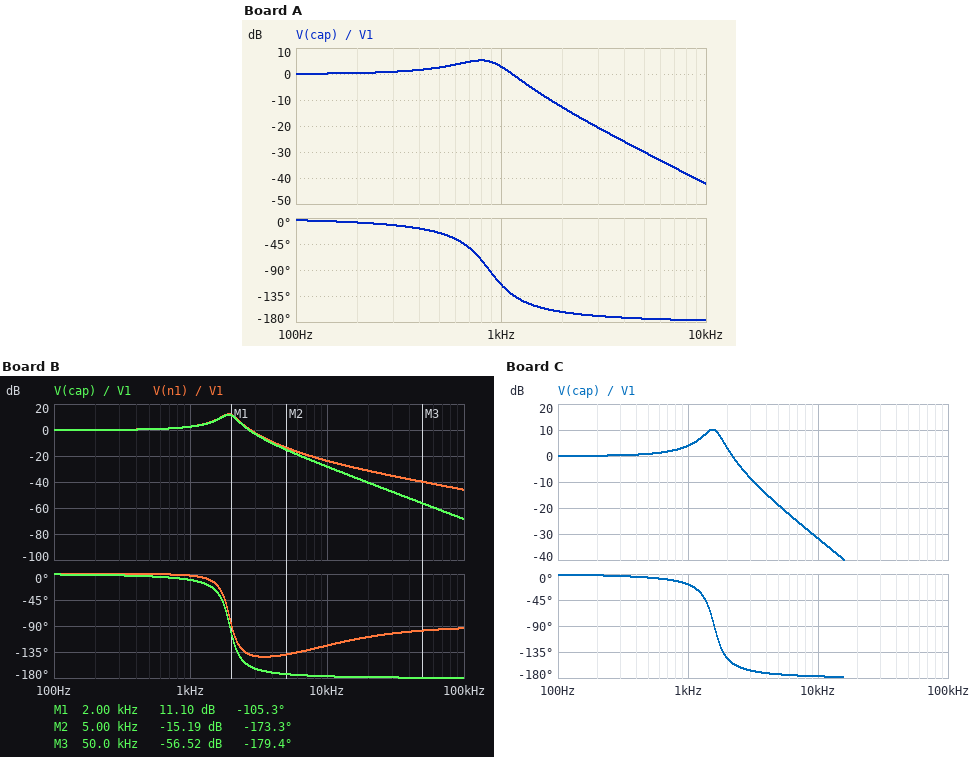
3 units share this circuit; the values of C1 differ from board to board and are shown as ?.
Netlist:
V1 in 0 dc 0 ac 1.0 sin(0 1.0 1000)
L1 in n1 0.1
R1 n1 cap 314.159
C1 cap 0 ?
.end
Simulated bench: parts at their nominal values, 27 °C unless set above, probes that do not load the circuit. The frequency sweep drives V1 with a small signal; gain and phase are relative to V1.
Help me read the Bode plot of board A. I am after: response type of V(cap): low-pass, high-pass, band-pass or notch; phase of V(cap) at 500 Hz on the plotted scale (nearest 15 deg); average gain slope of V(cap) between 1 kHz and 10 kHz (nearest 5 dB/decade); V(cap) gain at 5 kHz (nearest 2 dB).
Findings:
low-pass
-30 deg
-45 dB/decade
-30 dB
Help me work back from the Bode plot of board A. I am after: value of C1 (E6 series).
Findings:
330 nF
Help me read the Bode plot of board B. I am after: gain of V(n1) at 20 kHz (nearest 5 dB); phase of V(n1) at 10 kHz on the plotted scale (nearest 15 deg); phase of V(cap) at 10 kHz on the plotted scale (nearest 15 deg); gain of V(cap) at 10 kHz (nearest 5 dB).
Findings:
-30 dB
-120 deg
-180 deg
-30 dB
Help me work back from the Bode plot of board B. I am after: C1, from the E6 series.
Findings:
68 nF
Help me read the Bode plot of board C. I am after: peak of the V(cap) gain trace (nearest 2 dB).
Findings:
10 dB
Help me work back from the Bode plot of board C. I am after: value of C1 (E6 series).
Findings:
100 nF
